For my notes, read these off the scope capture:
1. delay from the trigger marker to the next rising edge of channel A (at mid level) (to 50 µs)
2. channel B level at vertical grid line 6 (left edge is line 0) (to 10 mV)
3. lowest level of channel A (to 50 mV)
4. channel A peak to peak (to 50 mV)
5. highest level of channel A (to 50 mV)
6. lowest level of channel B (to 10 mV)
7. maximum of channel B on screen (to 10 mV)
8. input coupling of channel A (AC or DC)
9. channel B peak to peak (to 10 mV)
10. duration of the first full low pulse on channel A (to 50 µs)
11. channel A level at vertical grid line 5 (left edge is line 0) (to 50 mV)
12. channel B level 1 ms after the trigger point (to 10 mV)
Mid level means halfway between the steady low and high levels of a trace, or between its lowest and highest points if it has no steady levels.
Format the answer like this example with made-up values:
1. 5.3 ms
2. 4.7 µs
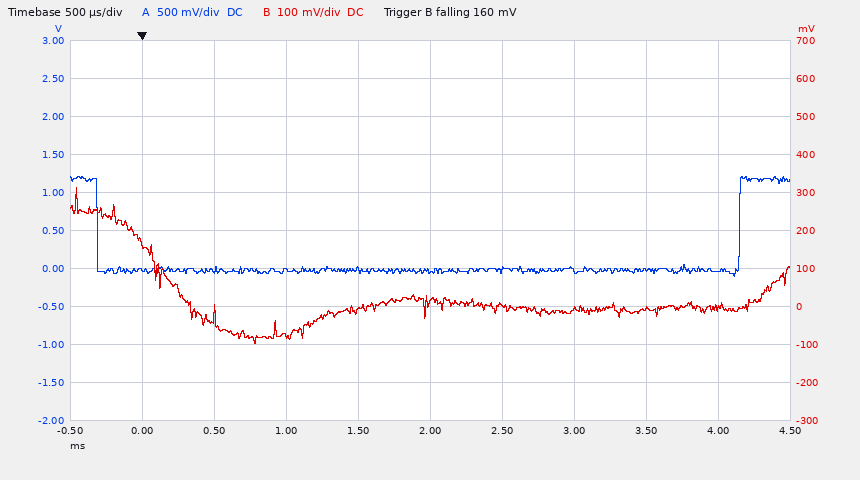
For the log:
1. 4.15 ms
2. 0 mV
3. -100 mV
4. 1.30 V
5. 1.20 V
6. -100 mV
7. 310 mV
8. DC
9. 410 mV
10. 4.45 ms
11. -50 mV
12. -80 mV
